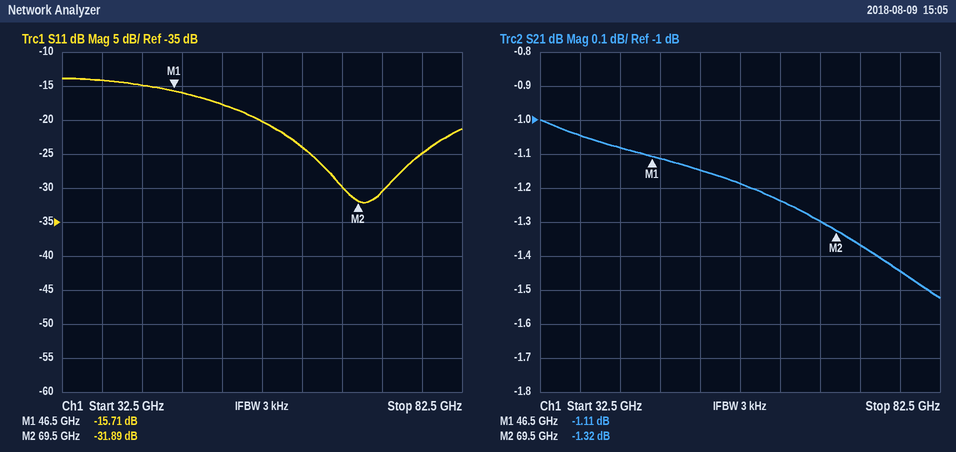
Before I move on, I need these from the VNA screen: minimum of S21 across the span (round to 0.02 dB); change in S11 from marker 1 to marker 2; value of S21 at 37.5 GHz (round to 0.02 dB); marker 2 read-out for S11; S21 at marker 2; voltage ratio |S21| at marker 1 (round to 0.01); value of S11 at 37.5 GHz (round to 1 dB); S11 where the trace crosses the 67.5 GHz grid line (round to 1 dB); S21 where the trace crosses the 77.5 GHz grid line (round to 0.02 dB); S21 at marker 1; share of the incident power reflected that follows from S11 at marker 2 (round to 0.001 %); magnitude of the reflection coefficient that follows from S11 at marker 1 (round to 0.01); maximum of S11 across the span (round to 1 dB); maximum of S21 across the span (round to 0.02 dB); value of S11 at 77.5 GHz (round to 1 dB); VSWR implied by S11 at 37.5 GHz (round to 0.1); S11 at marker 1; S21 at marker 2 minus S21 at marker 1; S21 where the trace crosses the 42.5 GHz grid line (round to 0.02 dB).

-1.52 dB
-16.18 dB
-1.04 dB
-31.89 dB
-1.32 dB
0.88
-14 dB
-30 dB
-1.44 dB
-1.11 dB
0.065 %
0.16
-14 dB
-1.00 dB
-25 dB
1.5
-15.71 dB
-0.21 dB
-1.08 dB
